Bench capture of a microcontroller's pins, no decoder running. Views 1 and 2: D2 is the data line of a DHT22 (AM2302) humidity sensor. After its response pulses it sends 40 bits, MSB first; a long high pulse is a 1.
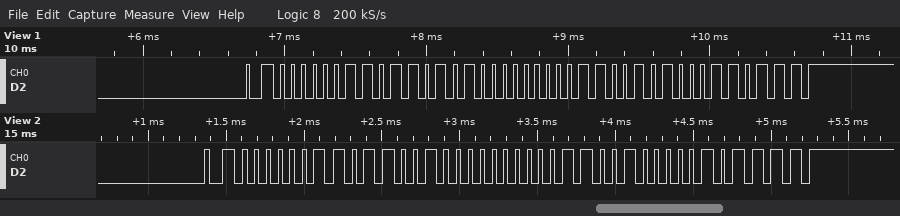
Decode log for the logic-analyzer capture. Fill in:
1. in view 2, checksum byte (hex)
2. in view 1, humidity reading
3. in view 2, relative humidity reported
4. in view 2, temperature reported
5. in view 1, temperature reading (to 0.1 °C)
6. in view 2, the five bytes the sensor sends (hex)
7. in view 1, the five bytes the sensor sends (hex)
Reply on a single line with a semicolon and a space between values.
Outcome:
0x2F; 87.4 %; 86.8 %; 20.0 °C; 20.2 °C; 03 64 00 C8 2F; 03 6A 00 CA 37
